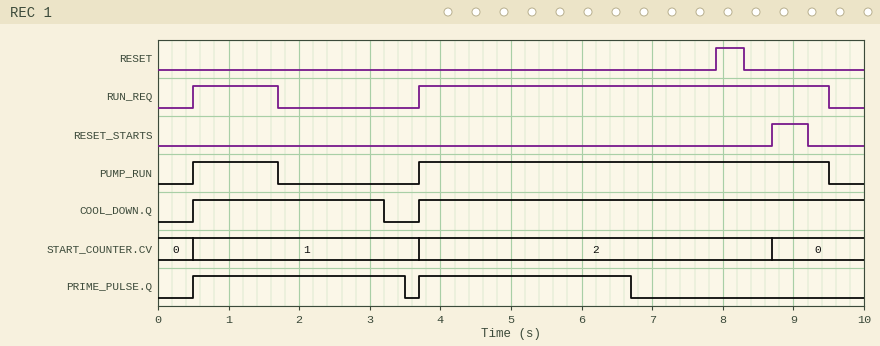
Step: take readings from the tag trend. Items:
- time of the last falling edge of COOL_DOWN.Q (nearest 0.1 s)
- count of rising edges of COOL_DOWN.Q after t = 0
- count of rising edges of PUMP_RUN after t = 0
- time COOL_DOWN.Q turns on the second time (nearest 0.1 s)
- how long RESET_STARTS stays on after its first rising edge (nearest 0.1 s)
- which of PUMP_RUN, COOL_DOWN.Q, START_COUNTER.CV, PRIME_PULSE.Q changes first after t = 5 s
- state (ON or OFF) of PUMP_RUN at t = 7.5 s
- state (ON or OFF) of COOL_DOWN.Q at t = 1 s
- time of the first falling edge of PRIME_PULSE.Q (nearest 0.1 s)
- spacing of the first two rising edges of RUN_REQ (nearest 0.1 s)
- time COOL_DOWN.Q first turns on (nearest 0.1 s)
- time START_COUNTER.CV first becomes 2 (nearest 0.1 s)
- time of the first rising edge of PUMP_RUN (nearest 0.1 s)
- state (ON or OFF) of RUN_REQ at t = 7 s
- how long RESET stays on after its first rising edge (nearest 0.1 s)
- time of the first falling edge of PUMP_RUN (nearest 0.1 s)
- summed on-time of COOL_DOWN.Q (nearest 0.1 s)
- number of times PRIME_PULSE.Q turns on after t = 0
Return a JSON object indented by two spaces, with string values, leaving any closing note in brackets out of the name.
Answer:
{
  "time of the last falling edge of COOL_DOWN.Q": "3.2 s",
  "count of rising edges of COOL_DOWN.Q after t = 0": "2",
  "count of rising edges of PUMP_RUN after t = 0": "2",
  "time COOL_DOWN.Q turns on the second time": "3.7 s",
  "how long RESET_STARTS stays on after its first rising edge": "0.5 s",
  "which of PUMP_RUN, COOL_DOWN.Q, START_COUNTER.CV, PRIME_PULSE.Q changes first after t = 5 s": "PRIME_PULSE.Q",
  "state (ON or OFF) of PUMP_RUN at t = 7.5 s": "ON",
  "state (ON or OFF) of COOL_DOWN.Q at t = 1 s": "ON",
  "time of the first falling edge of PRIME_PULSE.Q": "3.5 s",
  "spacing of the first two rising edges of RUN_REQ": "3.2 s",
  "time COOL_DOWN.Q first turns on": "0.5 s",
  "time START_COUNTER.CV first becomes 2": "3.7 s",
  "time of the first rising edge of PUMP_RUN": "0.5 s",
  "state (ON or OFF) of RUN_REQ at t = 7 s": "ON",
  "how long RESET stays on after its first rising edge": "0.4 s",
  "time of the first falling edge of PUMP_RUN": "1.7 s",
  "summed on-time of COOL_DOWN.Q": "9.0 s",
  "number of times PRIME_PULSE.Q turns on after t = 0": "2"
}
